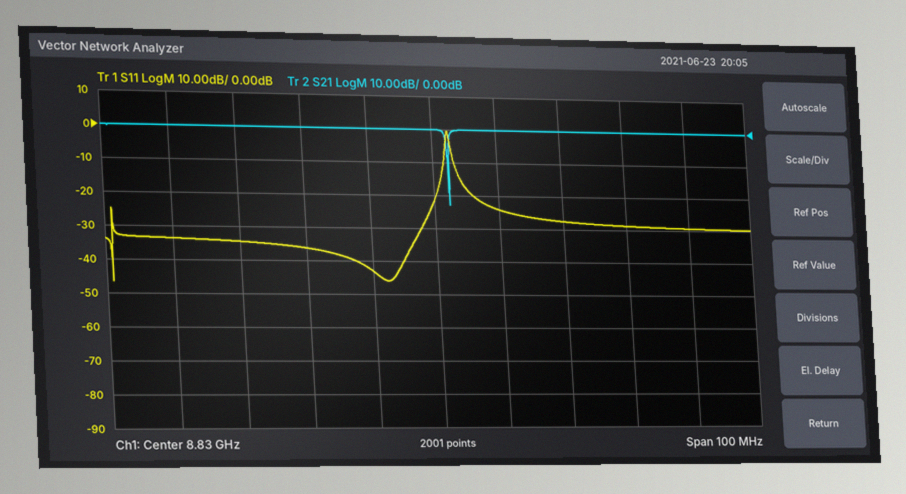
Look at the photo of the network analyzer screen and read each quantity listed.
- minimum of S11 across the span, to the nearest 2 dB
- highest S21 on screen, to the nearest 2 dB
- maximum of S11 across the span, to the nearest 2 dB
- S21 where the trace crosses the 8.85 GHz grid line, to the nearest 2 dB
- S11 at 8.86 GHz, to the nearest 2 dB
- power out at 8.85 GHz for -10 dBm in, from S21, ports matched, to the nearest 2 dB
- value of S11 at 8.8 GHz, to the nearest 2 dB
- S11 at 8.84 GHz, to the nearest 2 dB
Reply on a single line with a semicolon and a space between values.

-46 dB; 0 dB; 0 dB; 0 dB; -28 dB; -10 dBm; -34 dB; -24 dB
